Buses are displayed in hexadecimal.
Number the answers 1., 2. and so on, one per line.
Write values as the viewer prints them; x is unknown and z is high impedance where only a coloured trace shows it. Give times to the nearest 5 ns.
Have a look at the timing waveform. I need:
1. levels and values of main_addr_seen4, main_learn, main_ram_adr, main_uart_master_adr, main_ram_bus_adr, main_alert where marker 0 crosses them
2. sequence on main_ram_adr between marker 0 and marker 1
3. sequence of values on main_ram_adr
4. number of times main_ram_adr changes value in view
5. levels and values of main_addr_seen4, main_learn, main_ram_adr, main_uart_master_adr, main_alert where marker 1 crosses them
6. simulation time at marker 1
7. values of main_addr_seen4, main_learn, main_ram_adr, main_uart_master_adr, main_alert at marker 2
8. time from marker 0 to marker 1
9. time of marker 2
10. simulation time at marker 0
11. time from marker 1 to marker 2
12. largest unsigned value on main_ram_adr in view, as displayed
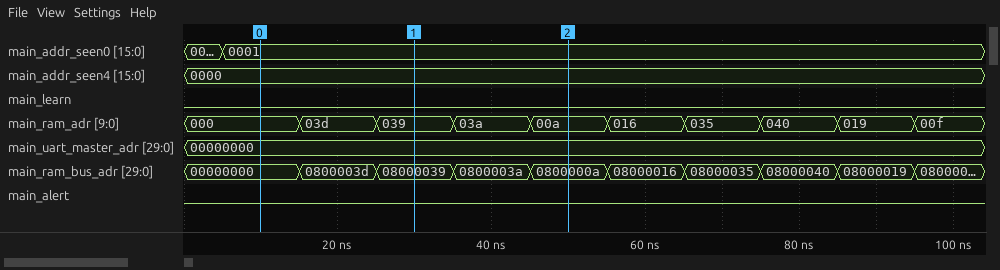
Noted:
1. main_addr_seen4=0000, main_learn=0, main_ram_adr=000, main_uart_master_adr=00000000, main_ram_bus_adr=00000000, main_alert=0
2. 000, 03d, 039
3. 000, 03d, 039, 03a, 00a, 016, 035, 040, 019, 00f
4. 9
5. main_addr_seen4=0000, main_learn=0, main_ram_adr=039, main_uart_master_adr=00000000, main_alert=0
6. 30 ns
7. main_addr_seen4=0000, main_learn=0, main_ram_adr=00a, main_uart_master_adr=00000000, main_alert=0
8. 20 ns
9. 50 ns
10. 10 ns
11. 20 ns
12. 040
